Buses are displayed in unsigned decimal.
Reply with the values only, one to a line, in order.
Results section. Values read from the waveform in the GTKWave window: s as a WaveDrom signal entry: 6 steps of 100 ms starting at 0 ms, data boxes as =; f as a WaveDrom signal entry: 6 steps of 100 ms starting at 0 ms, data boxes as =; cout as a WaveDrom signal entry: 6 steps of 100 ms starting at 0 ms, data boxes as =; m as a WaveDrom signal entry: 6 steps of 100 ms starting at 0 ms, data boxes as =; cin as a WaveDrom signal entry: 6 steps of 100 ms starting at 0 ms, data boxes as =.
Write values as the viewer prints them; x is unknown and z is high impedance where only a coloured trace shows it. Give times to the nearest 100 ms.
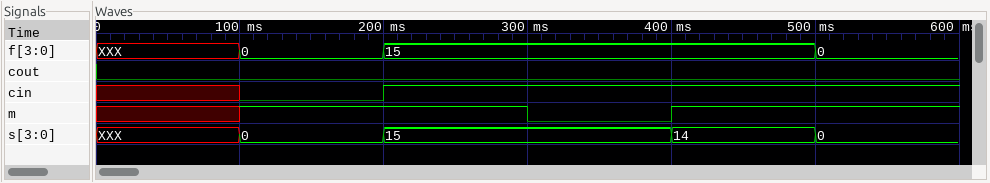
{name: 's', wave: 'x==.==', data: '0 15 14 0'}
{name: 'f', wave: 'x==..=', data: '0 15 0'}
{name: 'cout', wave: '0.....'}
{name: 'm', wave: 'x1.01.'}
{name: 'cin', wave: 'x01...'}
